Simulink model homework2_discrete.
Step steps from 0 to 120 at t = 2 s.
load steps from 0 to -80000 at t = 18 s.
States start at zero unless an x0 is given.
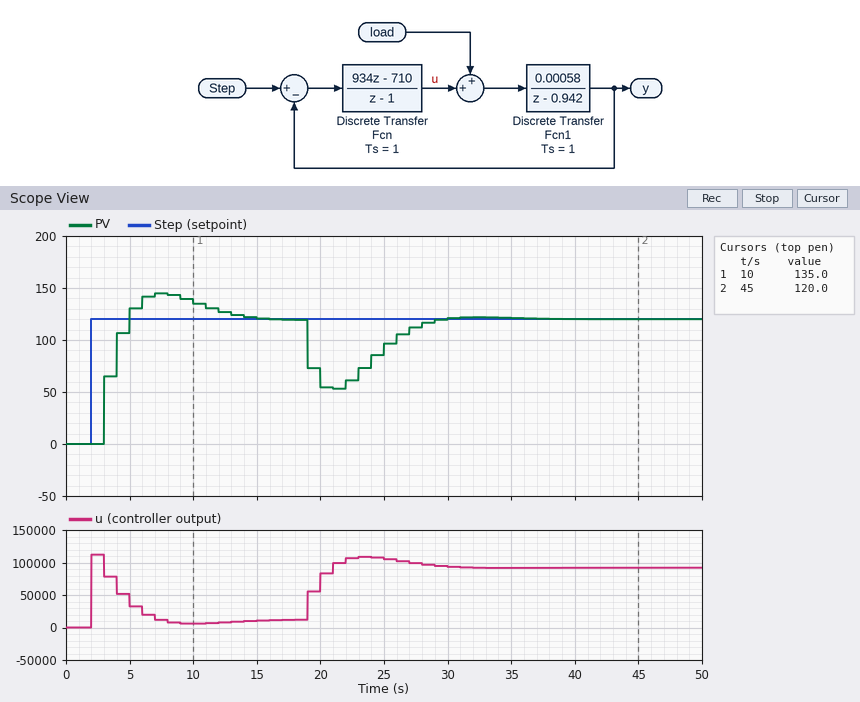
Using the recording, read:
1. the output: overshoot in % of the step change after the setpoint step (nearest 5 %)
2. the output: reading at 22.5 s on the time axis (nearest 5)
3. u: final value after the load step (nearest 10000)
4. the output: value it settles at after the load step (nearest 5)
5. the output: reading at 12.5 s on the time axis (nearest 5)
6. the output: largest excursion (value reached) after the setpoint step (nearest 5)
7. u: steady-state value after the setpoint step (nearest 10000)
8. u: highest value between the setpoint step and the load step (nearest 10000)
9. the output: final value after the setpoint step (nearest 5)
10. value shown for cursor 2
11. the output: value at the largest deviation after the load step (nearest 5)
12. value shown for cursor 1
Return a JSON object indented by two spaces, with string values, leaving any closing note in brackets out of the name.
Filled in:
{
  "the output: overshoot in % of the step change after the setpoint step": "20 %",
  "the output: reading at 22.5 s on the time axis": "60",
  "u: final value after the load step": "90000",
  "the output: value it settles at after the load step": "120",
  "the output: reading at 12.5 s on the time axis": "125",
  "the output: largest excursion (value reached) after the setpoint step": "145",
  "u: steady-state value after the setpoint step": "10000",
  "u: highest value between the setpoint step and the load step": "110000",
  "the output: final value after the setpoint step": "120",
  "value shown for cursor 2": "120.0",
  "the output: value at the largest deviation after the load step": "55",
  "value shown for cursor 1": "135.0"
}
